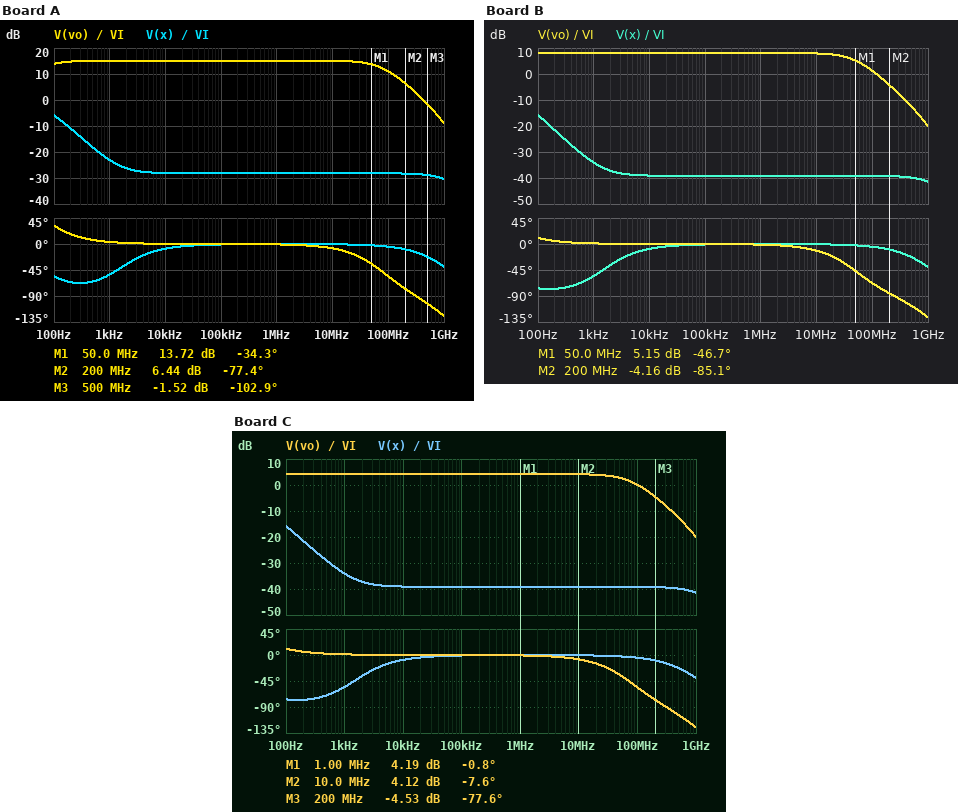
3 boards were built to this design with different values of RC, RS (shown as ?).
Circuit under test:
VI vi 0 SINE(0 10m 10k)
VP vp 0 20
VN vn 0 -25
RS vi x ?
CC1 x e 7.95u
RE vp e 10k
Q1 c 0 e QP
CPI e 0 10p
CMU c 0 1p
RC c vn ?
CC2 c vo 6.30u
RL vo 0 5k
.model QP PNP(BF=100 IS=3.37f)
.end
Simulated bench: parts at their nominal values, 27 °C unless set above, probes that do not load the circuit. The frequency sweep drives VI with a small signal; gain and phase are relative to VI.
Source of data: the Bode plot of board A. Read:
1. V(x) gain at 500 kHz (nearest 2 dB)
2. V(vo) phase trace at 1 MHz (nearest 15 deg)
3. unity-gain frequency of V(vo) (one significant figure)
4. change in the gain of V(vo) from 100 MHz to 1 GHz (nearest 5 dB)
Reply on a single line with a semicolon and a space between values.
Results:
-28 dB; 0 deg; 400 MHz; -20 dB
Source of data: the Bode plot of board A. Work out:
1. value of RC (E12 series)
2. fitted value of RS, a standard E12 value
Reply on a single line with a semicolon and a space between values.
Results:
3.3 kΩ; 330 Ω
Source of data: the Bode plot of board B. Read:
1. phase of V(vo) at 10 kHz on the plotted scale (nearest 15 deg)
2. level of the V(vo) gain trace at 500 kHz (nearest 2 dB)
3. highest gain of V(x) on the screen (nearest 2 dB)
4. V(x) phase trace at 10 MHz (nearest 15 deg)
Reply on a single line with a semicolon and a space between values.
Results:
0 deg; 8 dB; -16 dB; 0 deg
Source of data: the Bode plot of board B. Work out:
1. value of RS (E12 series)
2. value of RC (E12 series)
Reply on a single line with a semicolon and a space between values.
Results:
1.2 kΩ; 8.2 kΩ
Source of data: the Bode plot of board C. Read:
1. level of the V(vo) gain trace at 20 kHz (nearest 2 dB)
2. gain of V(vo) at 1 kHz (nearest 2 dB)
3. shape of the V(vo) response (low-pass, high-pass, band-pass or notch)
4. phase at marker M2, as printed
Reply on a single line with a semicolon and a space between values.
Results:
4 dB; 4 dB; low-pass; -7.6 deg
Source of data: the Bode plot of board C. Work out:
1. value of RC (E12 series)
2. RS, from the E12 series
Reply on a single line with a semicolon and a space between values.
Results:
3.3 kΩ; 1.2 kΩ
